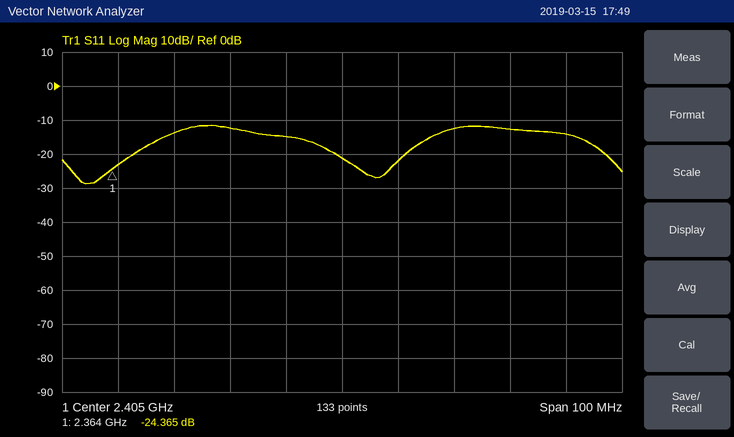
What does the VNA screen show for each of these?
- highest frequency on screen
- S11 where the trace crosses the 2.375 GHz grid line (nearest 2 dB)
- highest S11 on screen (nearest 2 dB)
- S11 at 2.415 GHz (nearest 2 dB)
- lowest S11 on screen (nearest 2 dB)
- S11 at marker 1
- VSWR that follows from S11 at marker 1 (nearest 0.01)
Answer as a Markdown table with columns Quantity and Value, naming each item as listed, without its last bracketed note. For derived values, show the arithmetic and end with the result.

| Quantity | Value |
|---|---|
| highest frequency on screen | 2.455 GHz |
| S11 where the trace crosses the 2.375 GHz grid line | -14 dB |
| highest S11 on screen | -12 dB |
| S11 at 2.415 GHz | -22 dB |
| lowest S11 on screen | -28 dB |
| S11 at marker 1 | -24.365 dB |
| VSWR that follows from S11 at marker 1 | (1 + 0.0605)/(1 − 0.0605) ≈ 1.13 |
